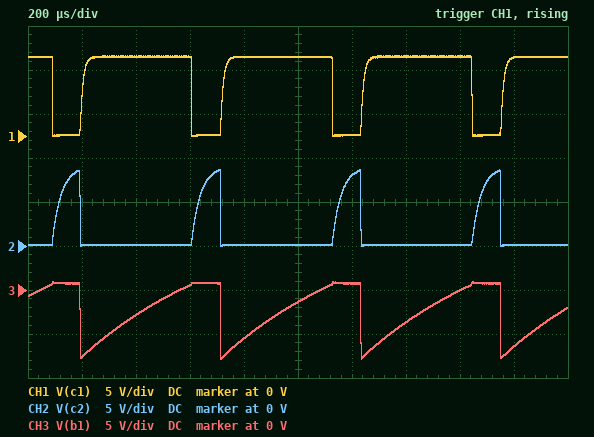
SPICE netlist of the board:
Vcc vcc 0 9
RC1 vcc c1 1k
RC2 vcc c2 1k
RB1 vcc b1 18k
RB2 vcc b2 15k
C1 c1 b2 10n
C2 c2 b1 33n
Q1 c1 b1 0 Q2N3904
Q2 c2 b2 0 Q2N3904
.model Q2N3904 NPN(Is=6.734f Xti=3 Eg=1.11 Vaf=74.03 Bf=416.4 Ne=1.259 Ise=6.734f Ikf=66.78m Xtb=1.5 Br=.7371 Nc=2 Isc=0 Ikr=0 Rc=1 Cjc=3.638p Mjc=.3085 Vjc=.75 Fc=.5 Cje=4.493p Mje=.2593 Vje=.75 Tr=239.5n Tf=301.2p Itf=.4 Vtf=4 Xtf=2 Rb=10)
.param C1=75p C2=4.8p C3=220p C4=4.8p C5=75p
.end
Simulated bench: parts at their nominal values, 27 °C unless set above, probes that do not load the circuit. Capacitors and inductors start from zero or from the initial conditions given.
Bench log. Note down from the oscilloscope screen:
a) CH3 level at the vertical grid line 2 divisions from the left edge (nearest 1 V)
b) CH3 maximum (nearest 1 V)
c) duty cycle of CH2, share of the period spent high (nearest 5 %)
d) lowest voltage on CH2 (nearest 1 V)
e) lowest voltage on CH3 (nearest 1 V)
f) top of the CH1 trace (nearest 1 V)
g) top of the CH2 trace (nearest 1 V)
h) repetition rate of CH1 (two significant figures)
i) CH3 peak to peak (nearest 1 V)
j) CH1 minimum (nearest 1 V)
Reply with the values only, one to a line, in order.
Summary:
-3 V
1 V
15 %
0 V
-8 V
9 V
9 V
1.9 kHz
9 V
0 V
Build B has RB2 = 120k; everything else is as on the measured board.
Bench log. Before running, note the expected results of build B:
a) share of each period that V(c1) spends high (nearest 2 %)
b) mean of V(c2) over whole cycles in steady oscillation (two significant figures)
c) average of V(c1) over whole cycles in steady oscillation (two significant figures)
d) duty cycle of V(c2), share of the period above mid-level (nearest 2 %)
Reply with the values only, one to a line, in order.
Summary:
32 %
5.9 V
2.9 V
66 %
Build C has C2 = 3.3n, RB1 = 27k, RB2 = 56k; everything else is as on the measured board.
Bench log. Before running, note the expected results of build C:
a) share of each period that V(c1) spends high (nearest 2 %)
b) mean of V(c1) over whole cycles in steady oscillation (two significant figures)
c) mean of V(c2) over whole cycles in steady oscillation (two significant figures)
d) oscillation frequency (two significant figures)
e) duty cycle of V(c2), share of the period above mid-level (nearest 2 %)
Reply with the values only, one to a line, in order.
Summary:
12 %
1.1 V
7.7 V
2.2 kHz
86 %
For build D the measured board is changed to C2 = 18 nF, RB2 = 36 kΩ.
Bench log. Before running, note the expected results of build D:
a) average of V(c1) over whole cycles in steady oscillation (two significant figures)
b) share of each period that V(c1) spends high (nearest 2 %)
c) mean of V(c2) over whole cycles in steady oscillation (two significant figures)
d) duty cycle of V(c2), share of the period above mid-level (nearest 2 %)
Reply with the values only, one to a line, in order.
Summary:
4.1 V
46 %
4.5 V
50 %
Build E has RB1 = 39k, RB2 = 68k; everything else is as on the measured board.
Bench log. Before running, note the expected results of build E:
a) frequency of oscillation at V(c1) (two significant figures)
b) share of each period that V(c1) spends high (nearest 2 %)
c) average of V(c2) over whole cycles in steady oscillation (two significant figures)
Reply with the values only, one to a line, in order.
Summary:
720 Hz
64 %
3.0 V
